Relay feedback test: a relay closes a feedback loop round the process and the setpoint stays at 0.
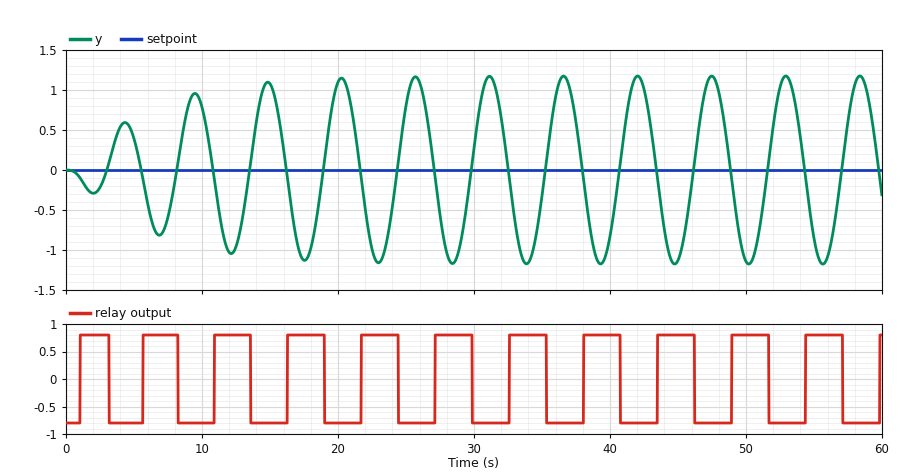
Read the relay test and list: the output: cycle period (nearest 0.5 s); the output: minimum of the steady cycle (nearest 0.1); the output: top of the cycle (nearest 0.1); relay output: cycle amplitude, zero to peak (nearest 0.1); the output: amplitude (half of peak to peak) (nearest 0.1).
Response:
5.5 s
-1.2
1.2
0.8
1.2
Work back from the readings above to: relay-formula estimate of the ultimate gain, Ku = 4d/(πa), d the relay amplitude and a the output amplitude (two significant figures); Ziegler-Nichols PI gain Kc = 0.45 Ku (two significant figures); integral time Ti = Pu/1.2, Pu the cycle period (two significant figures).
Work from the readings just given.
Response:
0.85
0.38
4.6 s
